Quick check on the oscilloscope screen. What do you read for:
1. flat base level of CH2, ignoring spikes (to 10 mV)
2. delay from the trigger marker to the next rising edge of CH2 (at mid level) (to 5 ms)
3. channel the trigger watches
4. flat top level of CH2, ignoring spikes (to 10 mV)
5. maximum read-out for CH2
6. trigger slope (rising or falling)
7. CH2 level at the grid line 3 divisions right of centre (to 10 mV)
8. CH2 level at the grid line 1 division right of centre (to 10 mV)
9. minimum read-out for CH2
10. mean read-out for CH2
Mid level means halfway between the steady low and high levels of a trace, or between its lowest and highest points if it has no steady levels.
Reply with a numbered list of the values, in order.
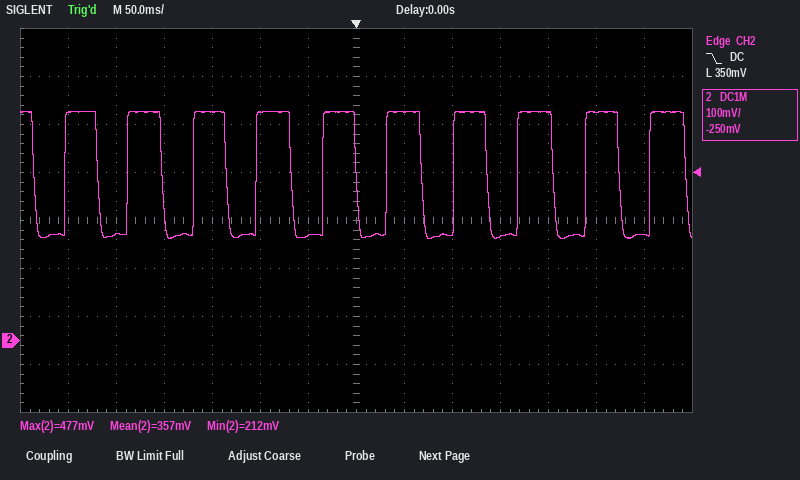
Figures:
1. 220 mV
2. 30 ms
3. CH2
4. 480 mV
5. 477 mV
6. falling
7. 220 mV
8. 480 mV
9. 212 mV
10. 357 mV
